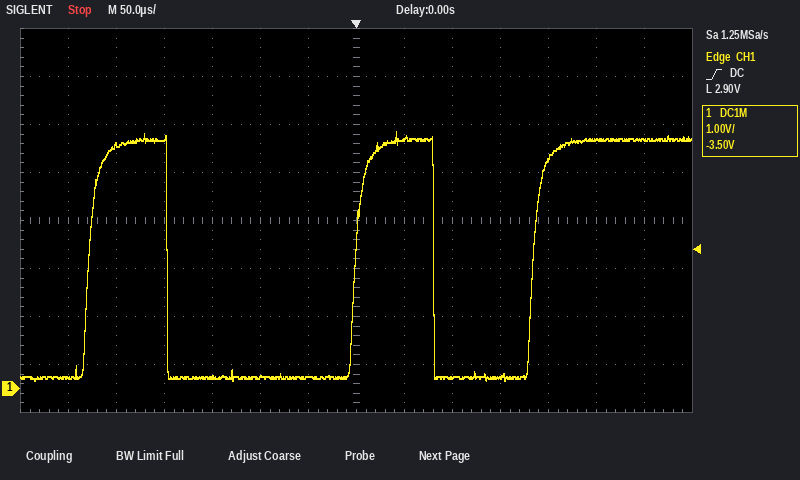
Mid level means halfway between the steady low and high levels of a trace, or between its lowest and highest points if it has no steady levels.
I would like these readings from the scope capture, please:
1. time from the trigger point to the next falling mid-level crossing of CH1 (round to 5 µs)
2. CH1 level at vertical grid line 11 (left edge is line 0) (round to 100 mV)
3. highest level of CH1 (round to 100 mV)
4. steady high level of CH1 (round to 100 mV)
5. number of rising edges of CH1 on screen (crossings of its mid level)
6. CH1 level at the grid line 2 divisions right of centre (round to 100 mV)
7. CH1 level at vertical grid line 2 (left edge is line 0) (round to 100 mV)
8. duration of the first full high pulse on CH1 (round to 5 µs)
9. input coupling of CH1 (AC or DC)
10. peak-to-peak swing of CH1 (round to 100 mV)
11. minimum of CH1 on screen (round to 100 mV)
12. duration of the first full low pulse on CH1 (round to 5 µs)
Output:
80 µs
4.8 V
5.4 V
5.2 V
3
200 mV
5.1 V
80 µs
DC
5.2 V
200 mV
195 µs
